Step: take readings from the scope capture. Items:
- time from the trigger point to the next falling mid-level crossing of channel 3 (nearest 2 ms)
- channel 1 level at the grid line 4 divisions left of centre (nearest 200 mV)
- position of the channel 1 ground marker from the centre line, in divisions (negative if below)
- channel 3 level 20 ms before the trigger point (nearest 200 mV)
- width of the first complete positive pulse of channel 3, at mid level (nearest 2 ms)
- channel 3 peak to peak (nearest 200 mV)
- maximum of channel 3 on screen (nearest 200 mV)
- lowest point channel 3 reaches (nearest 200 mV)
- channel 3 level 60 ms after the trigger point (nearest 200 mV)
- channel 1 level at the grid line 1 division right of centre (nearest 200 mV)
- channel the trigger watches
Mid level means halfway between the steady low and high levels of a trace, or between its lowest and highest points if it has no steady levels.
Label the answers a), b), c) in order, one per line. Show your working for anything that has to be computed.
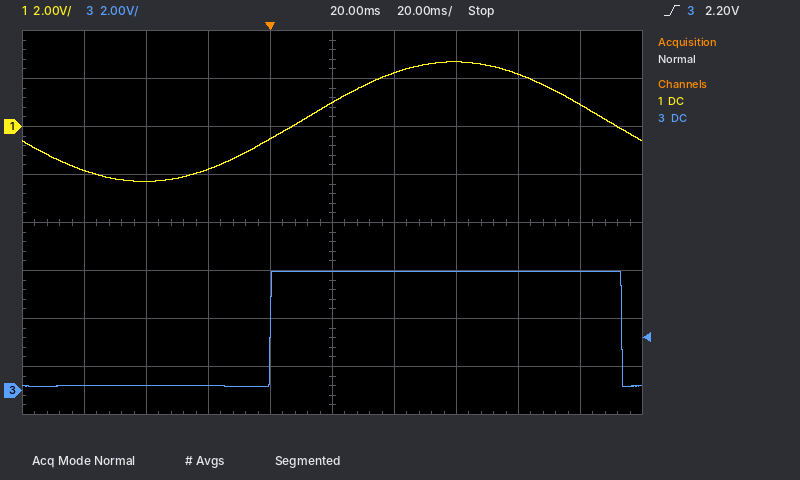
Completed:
a) 114 ms
b) -1.8 V
c) +2.0 div
d) 200 mV
e) 114 ms
f) 5.0 V − (200 mV) = 4.8 V
g) 5.0 V
h) 200 mV
i) 5.0 V
j) 2.2 V
k) channel 3
